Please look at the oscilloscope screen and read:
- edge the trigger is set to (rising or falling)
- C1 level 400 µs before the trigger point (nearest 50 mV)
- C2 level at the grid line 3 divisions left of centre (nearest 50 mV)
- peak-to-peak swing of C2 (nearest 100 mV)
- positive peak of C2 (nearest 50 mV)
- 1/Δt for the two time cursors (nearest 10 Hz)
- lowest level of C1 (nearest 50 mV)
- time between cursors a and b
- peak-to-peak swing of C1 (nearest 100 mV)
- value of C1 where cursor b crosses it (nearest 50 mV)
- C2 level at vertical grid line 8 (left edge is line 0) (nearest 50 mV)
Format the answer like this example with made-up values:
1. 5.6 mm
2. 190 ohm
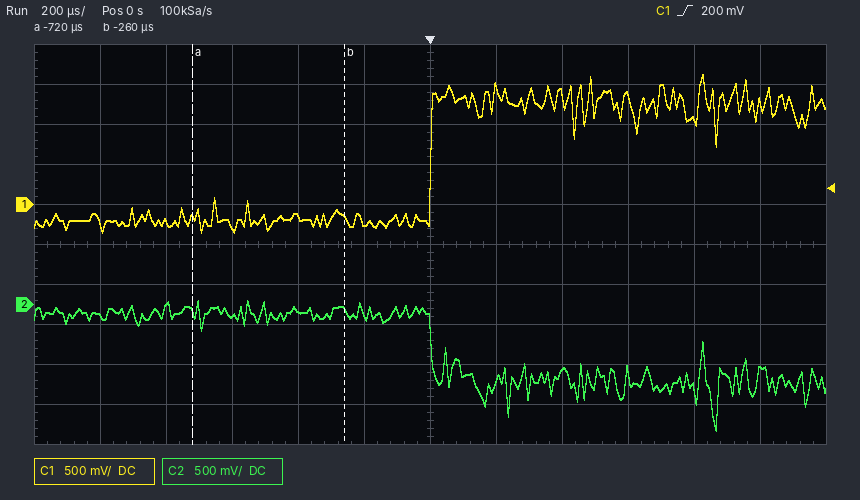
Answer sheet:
1. rising
2. -150 mV
3. -150 mV
4. 1.60 V
5. 50 mV
6. 2.17 kHz
7. -350 mV
8. 460 µs
9. 2.00 V
10. -150 mV
11. -850 mV
